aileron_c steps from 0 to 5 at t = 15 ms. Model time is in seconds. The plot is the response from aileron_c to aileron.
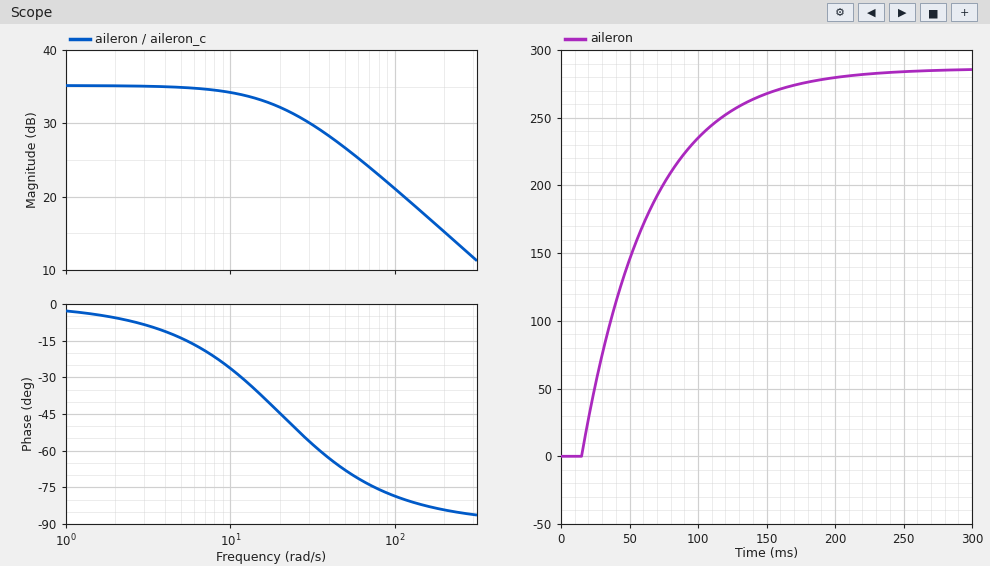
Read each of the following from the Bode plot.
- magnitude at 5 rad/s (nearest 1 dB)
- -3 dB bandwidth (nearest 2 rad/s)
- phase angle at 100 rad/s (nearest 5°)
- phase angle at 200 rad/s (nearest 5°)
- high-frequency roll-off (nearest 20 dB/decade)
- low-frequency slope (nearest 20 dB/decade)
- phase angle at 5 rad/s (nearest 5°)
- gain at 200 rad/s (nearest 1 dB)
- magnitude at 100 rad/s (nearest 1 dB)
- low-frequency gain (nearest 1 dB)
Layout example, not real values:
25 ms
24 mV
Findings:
35 dB
20 rad/s
-80°
-85°
-20 dB/decade
0 dB/decade
-15°
15 dB
21 dB
35 dB
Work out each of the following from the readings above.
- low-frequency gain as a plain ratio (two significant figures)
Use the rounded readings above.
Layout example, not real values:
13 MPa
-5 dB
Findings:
56
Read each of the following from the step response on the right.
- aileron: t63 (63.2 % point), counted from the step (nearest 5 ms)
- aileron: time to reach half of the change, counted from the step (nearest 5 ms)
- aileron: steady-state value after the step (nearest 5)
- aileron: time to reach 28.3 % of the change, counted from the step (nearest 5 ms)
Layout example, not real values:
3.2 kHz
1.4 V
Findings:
50 ms
35 ms
285
15 ms
